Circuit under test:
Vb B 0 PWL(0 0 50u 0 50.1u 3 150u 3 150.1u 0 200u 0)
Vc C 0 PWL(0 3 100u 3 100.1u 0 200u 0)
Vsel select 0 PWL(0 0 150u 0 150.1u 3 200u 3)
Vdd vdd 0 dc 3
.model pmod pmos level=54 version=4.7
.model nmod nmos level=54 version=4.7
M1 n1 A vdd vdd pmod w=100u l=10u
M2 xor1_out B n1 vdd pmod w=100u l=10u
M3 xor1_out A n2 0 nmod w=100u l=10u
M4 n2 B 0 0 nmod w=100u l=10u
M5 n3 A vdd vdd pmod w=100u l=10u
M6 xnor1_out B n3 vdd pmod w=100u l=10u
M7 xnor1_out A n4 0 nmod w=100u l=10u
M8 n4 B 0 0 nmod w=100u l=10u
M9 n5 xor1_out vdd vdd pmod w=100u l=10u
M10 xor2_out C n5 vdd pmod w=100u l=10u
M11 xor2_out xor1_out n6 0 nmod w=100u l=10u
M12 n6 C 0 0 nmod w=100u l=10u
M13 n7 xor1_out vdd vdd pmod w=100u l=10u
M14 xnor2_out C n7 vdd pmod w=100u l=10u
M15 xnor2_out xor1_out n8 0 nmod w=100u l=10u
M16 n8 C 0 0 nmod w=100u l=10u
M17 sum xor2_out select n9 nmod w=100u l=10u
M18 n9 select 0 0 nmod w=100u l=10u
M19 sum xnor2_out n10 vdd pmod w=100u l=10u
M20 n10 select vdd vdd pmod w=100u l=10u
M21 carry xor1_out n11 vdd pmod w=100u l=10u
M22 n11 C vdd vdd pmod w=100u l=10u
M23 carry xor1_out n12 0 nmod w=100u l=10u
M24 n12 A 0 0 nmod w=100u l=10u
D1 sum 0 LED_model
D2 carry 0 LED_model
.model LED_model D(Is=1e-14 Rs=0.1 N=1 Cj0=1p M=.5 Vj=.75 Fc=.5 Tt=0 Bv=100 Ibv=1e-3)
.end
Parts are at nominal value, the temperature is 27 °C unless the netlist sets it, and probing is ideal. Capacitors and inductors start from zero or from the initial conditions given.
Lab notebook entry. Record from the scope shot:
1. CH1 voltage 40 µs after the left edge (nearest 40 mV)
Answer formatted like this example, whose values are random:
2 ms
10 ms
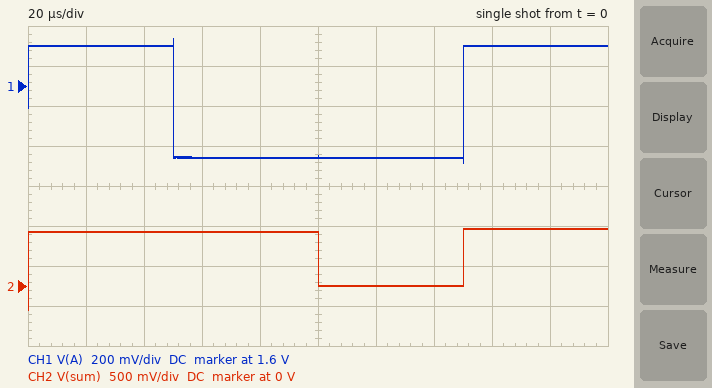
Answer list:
1.80 V
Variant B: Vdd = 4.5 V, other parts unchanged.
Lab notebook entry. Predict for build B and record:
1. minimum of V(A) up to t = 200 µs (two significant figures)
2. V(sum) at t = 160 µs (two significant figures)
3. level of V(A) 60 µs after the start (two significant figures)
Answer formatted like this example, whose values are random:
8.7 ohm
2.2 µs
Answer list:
1.8 V
730 mV
1.9 V
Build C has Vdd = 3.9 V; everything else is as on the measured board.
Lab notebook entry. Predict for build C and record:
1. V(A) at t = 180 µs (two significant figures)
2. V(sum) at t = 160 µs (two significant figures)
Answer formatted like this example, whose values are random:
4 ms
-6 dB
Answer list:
2.4 V
720 mV
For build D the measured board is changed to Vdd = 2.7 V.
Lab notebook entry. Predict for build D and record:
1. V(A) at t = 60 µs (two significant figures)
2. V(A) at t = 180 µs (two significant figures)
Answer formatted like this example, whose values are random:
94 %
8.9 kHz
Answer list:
1.1 V
1.6 V
